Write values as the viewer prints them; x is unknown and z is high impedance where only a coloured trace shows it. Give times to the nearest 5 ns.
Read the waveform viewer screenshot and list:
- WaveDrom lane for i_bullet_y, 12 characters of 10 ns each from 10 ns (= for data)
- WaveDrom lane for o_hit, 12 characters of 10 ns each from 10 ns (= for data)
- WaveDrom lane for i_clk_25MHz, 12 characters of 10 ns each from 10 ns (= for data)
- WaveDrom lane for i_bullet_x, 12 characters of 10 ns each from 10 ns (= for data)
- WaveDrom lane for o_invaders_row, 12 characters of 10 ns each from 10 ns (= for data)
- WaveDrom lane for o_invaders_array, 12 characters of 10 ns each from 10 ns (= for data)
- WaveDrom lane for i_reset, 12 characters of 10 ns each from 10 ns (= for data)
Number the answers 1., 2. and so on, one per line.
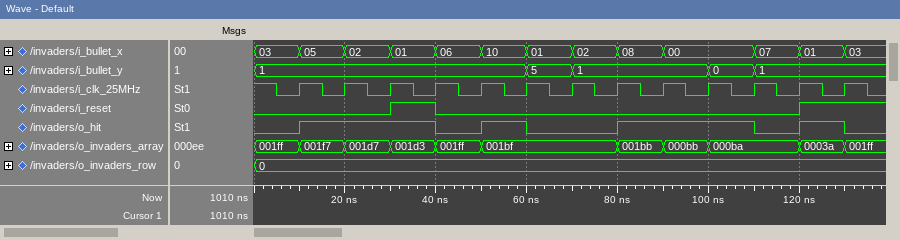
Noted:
1. {name: 'i_bullet_y', wave: '=....==..==.', data: '1 5 1 0 1'}
2. {name: 'o_hit', wave: '1..010.1..01'}
3. {name: 'i_clk_25MHz', wave: 'p...........'}
4. {name: 'i_bullet_x', wave: '=========.==', data: '05 02 01 06 10 01 02 08 00 07 01'}
5. {name: 'o_invaders_row', wave: '=...........', data: '0'}
6. {name: 'o_invaders_array', wave: '=====..===.=', data: '001f7 001d7 001d3 001ff 001bf 001bb 000bb 000ba 0003a'}
7. {name: 'i_reset', wave: '0.10.......1'}
